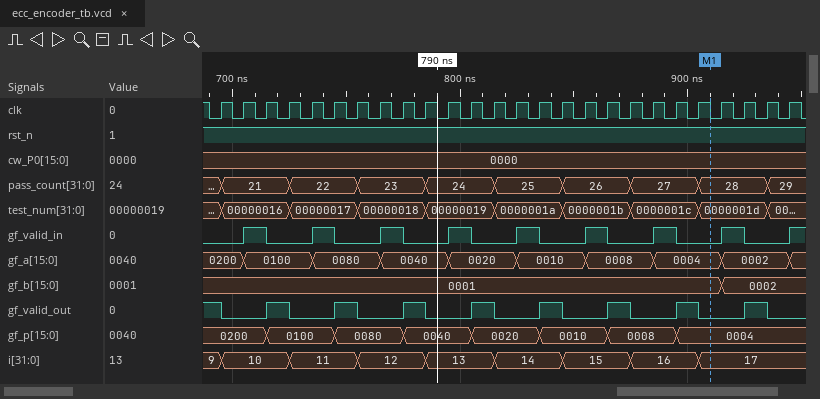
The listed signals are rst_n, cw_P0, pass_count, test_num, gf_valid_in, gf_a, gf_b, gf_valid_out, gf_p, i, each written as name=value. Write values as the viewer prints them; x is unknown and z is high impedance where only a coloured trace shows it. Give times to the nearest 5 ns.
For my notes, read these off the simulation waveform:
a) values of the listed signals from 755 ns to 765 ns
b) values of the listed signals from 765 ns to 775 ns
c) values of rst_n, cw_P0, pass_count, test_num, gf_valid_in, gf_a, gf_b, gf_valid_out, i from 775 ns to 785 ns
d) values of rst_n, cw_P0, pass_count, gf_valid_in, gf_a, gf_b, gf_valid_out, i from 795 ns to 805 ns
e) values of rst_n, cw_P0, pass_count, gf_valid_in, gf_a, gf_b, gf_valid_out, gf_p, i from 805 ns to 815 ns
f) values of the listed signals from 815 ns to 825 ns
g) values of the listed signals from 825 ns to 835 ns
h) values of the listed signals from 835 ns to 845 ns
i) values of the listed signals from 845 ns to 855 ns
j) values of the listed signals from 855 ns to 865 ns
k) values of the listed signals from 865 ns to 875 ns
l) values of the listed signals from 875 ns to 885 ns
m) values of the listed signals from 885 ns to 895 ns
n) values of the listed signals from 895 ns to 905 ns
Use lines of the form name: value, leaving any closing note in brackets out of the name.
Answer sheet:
values of the listed signals from 755 ns to 765 ns: rst_n=1, cw_P0=0000, pass_count=23, test_num=00000018, gf_valid_in=0, gf_a=0080, gf_b=0001, gf_valid_out=0, gf_p=0080, i=12
values of the listed signals from 765 ns to 775 ns: rst_n=1, cw_P0=0000, pass_count=23, test_num=00000018, gf_valid_in=1, gf_a=0040, gf_b=0001, gf_valid_out=0, gf_p=0080, i=12
values of rst_n, cw_P0, pass_count, test_num, gf_valid_in, gf_a, gf_b, gf_valid_out, i from 775 ns to 785 ns: rst_n=1, cw_P0=0000, pass_count=23, test_num=00000018, gf_valid_in=0, gf_a=0040, gf_b=0001, gf_valid_out=1, i=12
values of rst_n, cw_P0, pass_count, gf_valid_in, gf_a, gf_b, gf_valid_out, i from 795 ns to 805 ns: rst_n=1, cw_P0=0000, pass_count=24, gf_valid_in=1, gf_a=0020, gf_b=0001, gf_valid_out=0, i=13
values of rst_n, cw_P0, pass_count, gf_valid_in, gf_a, gf_b, gf_valid_out, gf_p, i from 805 ns to 815 ns: rst_n=1, cw_P0=0000, pass_count=24, gf_valid_in=0, gf_a=0020, gf_b=0001, gf_valid_out=1, gf_p=0020, i=13
values of the listed signals from 815 ns to 825 ns: rst_n=1, cw_P0=0000, pass_count=25, test_num=0000001a, gf_valid_in=0, gf_a=0020, gf_b=0001, gf_valid_out=0, gf_p=0020, i=14
values of the listed signals from 825 ns to 835 ns: rst_n=1, cw_P0=0000, pass_count=25, test_num=0000001a, gf_valid_in=1, gf_a=0010, gf_b=0001, gf_valid_out=0, gf_p=0020, i=14
values of the listed signals from 835 ns to 845 ns: rst_n=1, cw_P0=0000, pass_count=25, test_num=0000001a, gf_valid_in=0, gf_a=0010, gf_b=0001, gf_valid_out=1, gf_p=0010, i=14
values of the listed signals from 845 ns to 855 ns: rst_n=1, cw_P0=0000, pass_count=26, test_num=0000001b, gf_valid_in=0, gf_a=0010, gf_b=0001, gf_valid_out=0, gf_p=0010, i=15
values of the listed signals from 855 ns to 865 ns: rst_n=1, cw_P0=0000, pass_count=26, test_num=0000001b, gf_valid_in=1, gf_a=0008, gf_b=0001, gf_valid_out=0, gf_p=0010, i=15
values of the listed signals from 865 ns to 875 ns: rst_n=1, cw_P0=0000, pass_count=26, test_num=0000001b, gf_valid_in=0, gf_a=0008, gf_b=0001, gf_valid_out=1, gf_p=0008, i=15
values of the listed signals from 875 ns to 885 ns: rst_n=1, cw_P0=0000, pass_count=27, test_num=0000001c, gf_valid_in=0, gf_a=0008, gf_b=0001, gf_valid_out=0, gf_p=0008, i=16
values of the listed signals from 885 ns to 895 ns: rst_n=1, cw_P0=0000, pass_count=27, test_num=0000001c, gf_valid_in=1, gf_a=0004, gf_b=0001, gf_valid_out=0, gf_p=0008, i=16
values of the listed signals from 895 ns to 905 ns: rst_n=1, cw_P0=0000, pass_count=27, test_num=0000001c, gf_valid_in=0, gf_a=0004, gf_b=0001, gf_valid_out=1, gf_p=0004, i=16
